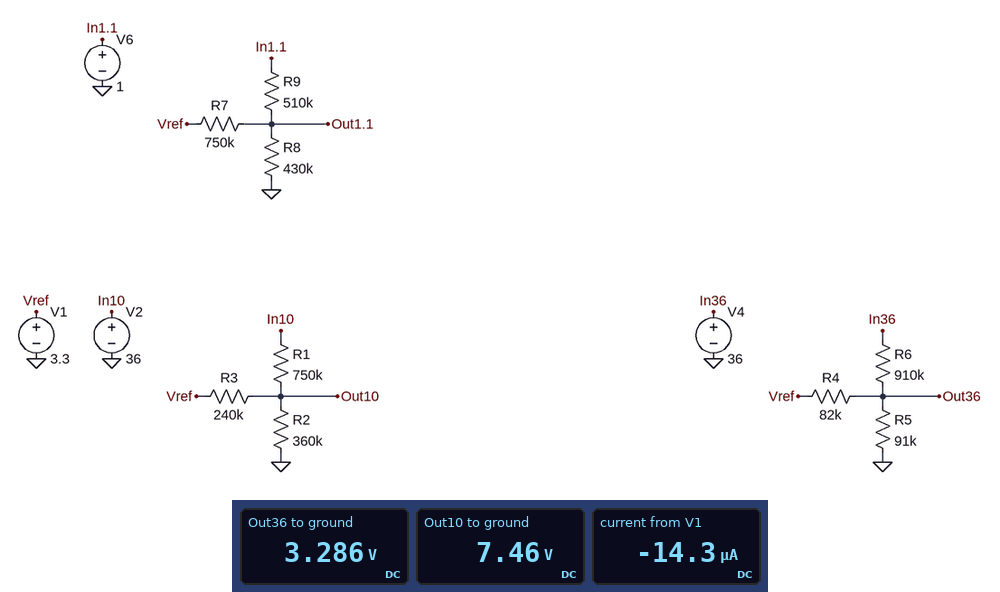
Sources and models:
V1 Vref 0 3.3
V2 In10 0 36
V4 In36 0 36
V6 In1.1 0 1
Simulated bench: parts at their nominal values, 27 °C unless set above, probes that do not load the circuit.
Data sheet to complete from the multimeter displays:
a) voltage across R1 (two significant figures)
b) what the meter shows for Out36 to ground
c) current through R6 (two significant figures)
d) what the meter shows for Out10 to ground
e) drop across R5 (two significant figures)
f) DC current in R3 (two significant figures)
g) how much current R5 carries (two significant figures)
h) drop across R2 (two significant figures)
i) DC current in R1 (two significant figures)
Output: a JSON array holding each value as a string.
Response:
["29 V", "3.286 V", "36 µA", "7.46 V", "3.3 V", "17 µA", "36 µA", "7.5 V", "38 µA"]
